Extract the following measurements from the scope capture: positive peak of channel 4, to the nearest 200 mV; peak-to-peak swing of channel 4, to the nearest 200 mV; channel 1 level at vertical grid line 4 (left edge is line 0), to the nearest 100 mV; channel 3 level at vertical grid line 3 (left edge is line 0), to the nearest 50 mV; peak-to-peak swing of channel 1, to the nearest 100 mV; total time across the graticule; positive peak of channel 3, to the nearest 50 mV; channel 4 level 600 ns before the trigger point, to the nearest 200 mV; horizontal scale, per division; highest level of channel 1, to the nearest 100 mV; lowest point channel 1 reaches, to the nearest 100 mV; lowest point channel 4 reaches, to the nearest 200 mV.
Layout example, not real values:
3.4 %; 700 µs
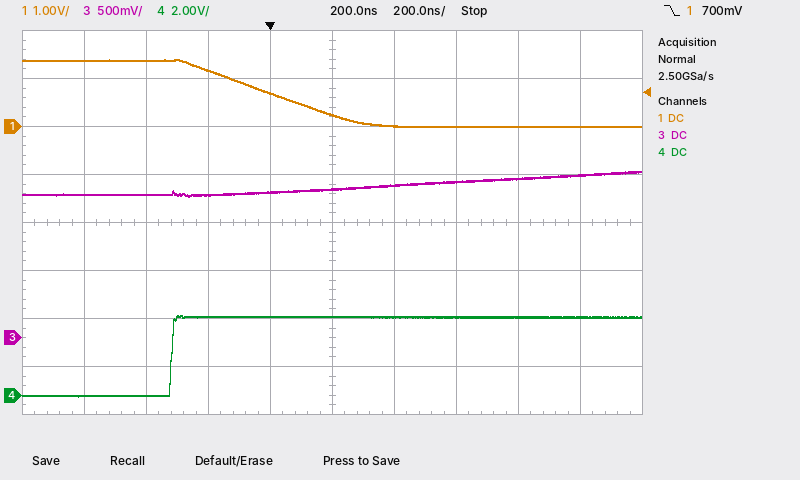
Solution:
3.4 V; 3.4 V; 700 mV; 1.50 V; 1.4 V; 2 µs; 1.75 V; 0.0 V; 200 ns; 1.4 V; 0.0 V; 0.0 V
